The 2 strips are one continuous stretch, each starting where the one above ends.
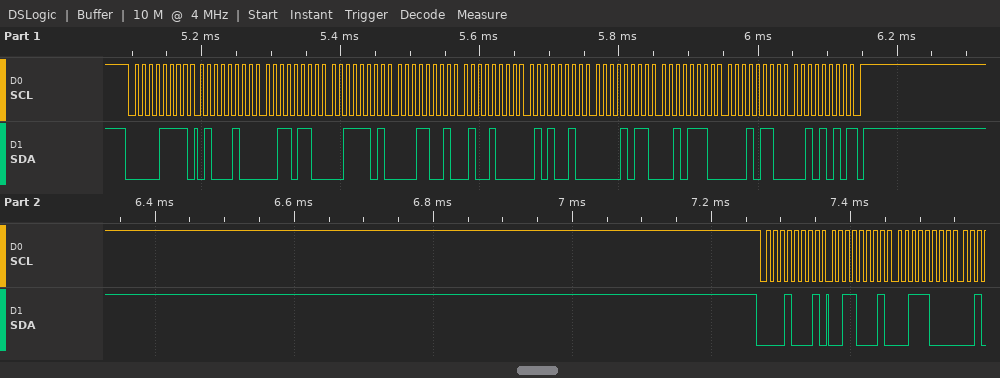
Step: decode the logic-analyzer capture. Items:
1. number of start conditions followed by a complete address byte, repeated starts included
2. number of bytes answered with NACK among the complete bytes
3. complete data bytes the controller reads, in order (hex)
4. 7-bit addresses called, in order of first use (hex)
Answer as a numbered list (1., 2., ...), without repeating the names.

1. 2
2. 1
3. 44 36 3D 19 48 52 0B 2E 16 2A 31 38
4. 0x07 0x08
